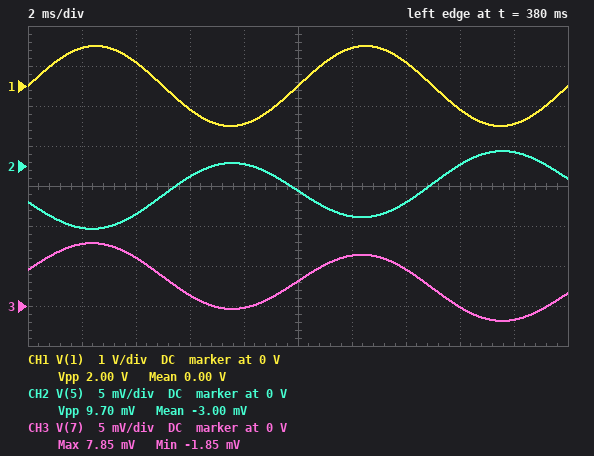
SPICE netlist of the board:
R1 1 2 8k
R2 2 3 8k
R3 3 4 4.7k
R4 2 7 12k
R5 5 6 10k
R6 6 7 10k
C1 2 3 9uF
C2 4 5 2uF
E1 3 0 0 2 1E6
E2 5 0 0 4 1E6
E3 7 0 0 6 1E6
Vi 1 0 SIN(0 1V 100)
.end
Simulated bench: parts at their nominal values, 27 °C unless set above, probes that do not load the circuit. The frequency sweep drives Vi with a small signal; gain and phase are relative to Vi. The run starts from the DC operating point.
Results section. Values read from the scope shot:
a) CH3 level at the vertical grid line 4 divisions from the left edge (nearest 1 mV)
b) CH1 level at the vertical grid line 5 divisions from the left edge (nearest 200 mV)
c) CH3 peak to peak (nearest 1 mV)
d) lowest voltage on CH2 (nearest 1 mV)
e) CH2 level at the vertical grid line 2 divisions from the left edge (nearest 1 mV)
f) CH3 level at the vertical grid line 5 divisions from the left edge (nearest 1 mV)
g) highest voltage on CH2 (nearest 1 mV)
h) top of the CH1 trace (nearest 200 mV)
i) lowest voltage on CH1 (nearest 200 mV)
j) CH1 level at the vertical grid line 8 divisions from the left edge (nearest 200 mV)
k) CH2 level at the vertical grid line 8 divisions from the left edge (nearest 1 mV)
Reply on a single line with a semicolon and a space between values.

0 V; 0 V; 10 mV; -8 mV; -6 mV; 3 mV; 2 mV; 1.0 V; -1.0 V; -600 mV; 0 V
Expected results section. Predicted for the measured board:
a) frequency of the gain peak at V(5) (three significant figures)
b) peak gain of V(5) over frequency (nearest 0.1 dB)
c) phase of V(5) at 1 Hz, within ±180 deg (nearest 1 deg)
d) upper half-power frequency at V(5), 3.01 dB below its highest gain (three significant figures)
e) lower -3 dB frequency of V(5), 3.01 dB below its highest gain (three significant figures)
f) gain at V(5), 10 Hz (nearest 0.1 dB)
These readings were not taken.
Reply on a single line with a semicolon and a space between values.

4.74 Hz; 10.8 dB; -5 deg; 5.77 Hz; 3.43 Hz; -6.4 dB
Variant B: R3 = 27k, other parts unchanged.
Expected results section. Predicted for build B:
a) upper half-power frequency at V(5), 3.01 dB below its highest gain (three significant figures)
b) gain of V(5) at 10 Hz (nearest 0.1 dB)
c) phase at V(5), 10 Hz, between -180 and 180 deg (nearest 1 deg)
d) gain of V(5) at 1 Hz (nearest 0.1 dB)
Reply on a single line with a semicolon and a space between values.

2.41 Hz; -23.6 dB; -167 deg; 4.2 dB
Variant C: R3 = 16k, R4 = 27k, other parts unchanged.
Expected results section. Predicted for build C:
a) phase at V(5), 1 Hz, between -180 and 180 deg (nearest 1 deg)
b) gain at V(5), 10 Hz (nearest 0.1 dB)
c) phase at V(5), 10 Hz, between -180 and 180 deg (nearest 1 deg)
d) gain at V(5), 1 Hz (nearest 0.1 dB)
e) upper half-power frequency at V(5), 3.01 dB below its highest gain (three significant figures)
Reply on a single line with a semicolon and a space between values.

-44 deg; -19.1 dB; -167 deg; 10.8 dB; 1.99 Hz
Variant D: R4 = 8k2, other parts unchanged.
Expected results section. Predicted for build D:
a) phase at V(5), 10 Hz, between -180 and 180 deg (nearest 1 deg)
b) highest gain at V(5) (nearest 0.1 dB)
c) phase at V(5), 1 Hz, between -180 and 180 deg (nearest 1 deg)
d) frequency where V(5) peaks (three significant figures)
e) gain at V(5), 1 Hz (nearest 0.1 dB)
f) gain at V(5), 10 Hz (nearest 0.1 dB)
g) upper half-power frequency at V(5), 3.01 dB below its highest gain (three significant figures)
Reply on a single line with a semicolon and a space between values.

-161 deg; 9.1 dB; -4 deg; 5.84 Hz; 0.4 dB; -5.1 dB; 6.87 Hz
